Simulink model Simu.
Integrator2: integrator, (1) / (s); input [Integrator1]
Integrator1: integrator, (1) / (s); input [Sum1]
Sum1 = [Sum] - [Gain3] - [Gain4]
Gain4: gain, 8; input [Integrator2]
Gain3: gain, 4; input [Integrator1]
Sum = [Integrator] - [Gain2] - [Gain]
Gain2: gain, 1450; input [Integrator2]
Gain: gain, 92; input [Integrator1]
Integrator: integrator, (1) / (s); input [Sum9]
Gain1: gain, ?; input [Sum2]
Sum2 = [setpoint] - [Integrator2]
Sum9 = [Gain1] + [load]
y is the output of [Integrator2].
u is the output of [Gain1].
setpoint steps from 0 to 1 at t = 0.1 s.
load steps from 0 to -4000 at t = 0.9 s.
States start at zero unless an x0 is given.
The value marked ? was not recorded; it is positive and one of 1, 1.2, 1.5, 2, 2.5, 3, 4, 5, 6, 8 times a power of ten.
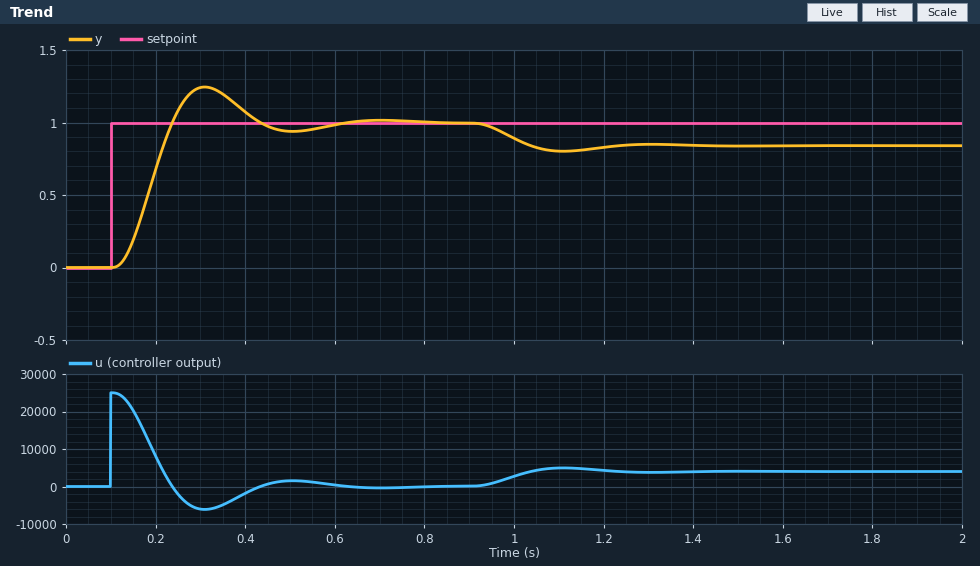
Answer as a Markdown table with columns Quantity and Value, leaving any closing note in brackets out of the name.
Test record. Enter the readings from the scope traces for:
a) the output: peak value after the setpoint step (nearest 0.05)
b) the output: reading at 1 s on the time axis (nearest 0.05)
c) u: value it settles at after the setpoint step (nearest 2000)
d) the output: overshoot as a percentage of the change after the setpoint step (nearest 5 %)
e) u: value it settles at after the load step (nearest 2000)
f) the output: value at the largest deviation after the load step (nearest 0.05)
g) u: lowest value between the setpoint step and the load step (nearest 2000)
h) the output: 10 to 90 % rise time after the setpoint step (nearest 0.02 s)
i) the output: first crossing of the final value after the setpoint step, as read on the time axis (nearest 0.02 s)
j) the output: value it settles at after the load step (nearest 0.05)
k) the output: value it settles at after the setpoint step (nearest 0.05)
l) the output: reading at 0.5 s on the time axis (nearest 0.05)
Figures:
| Quantity | Value |
|---|---|
| the output: peak value after the setpoint step | 1.25 |
| the output: reading at 1 s on the time axis | 0.90 |
| u: value it settles at after the setpoint step | 0 |
| the output: overshoot as a percentage of the change after the setpoint step | 25 % |
| u: value it settles at after the load step | 4000 |
| the output: value at the largest deviation after the load step | 0.80 |
| u: lowest value between the setpoint step and the load step | -6000 |
| the output: 10 to 90 % rise time after the setpoint step | 0.08 s |
| the output: first crossing of the final value after the setpoint step, as read on the time axis | 0.24 s |
| the output: value it settles at after the load step | 0.85 |
| the output: value it settles at after the setpoint step | 1.00 |
| the output: reading at 0.5 s on the time axis | 0.95 |
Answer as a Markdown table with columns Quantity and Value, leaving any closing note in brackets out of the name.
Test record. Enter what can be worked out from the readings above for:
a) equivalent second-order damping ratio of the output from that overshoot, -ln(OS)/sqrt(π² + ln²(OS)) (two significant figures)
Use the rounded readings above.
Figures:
| Quantity | Value |
|---|---|
| equivalent second-order damping ratio of the output from that overshoot, -ln(OS)/sqrt(π² + ln²(OS)) | 0.40 |
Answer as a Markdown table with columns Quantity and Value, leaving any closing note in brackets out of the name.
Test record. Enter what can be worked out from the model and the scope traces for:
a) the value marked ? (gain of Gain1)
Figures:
| Quantity | Value |
|---|---|
| the value marked ? | 25000 |
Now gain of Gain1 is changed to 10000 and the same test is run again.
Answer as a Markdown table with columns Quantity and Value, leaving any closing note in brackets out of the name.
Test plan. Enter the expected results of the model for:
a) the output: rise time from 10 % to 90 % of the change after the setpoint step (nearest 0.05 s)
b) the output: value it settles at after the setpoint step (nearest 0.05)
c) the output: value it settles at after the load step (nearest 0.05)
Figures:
| Quantity | Value |
|---|---|
| the output: rise time from 10 % to 90 % of the change after the setpoint step | 0.20 s |
| the output: value it settles at after the setpoint step | 1.00 |
| the output: value it settles at after the load step | 0.60 |
